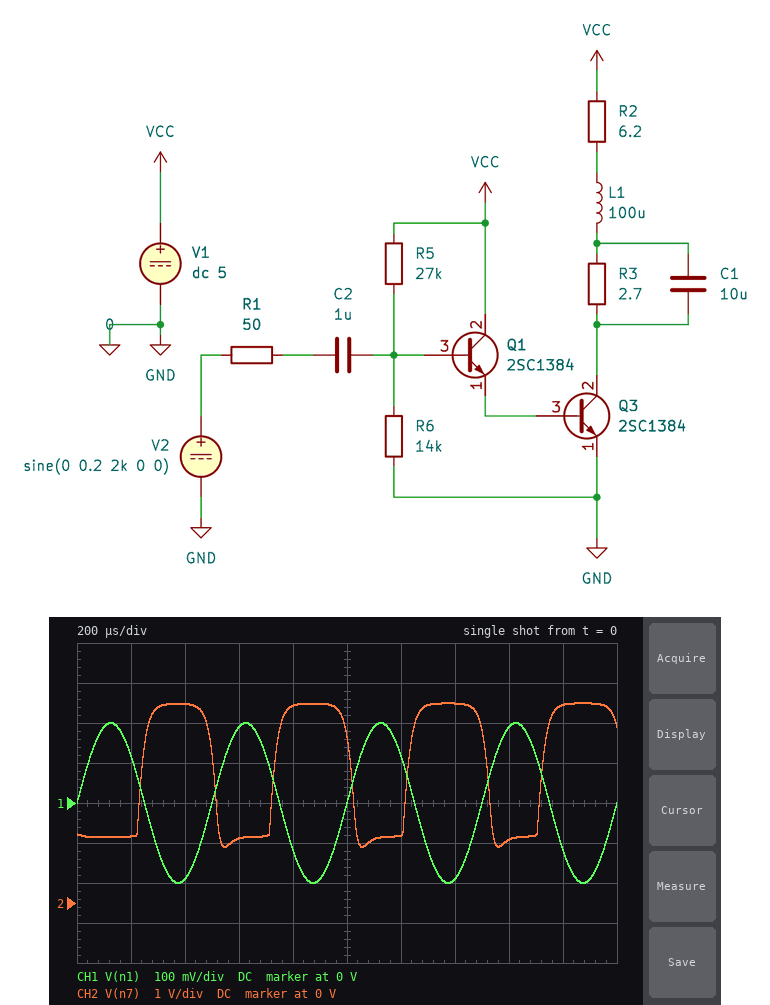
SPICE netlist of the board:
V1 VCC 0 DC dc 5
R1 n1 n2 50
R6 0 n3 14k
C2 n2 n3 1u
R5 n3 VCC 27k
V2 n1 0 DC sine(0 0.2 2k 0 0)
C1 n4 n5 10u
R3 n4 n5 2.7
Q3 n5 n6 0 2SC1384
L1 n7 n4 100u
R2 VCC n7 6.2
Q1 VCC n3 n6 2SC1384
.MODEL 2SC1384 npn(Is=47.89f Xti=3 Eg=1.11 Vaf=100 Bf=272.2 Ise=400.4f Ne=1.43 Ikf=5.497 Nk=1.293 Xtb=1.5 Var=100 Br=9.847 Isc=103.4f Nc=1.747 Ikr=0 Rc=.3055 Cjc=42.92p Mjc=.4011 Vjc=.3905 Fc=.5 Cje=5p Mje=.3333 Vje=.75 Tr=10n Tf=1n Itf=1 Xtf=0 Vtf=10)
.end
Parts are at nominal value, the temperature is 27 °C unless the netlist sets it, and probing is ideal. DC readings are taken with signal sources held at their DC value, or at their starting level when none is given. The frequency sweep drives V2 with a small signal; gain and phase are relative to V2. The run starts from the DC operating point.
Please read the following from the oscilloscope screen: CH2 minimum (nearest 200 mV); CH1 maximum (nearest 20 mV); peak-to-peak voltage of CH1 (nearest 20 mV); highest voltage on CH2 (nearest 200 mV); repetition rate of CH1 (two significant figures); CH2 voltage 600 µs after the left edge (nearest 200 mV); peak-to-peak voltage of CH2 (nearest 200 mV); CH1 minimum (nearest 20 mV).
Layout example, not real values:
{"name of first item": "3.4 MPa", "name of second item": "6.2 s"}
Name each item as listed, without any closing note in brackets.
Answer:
{"CH2 minimum": "1.4 V", "CH1 maximum": "200 mV", "peak-to-peak voltage of CH1": "400 mV", "highest voltage on CH2": "5.0 V", "repetition rate of CH1": "2.0 kHz", "CH2 voltage 600 µs after the left edge": "1.6 V", "peak-to-peak voltage of CH2": "3.6 V", "CH1 minimum": "-200 mV"}
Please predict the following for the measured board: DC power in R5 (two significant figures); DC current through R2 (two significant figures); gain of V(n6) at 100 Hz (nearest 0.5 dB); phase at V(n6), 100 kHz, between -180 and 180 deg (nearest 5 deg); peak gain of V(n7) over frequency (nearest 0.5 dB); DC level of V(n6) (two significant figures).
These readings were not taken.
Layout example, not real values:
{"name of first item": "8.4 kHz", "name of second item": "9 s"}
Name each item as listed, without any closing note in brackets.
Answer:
{"DC power in R5": "470 µW", "DC current through R2": "530 mA", "gain of V(n6) at 100 Hz": "-26.0 dB", "phase at V(n6), 100 kHz, between -180 and 180 deg": "-5 deg", "peak gain of V(n7) over frequency": "10.0 dB", "DC level of V(n6)": "780 mV"}
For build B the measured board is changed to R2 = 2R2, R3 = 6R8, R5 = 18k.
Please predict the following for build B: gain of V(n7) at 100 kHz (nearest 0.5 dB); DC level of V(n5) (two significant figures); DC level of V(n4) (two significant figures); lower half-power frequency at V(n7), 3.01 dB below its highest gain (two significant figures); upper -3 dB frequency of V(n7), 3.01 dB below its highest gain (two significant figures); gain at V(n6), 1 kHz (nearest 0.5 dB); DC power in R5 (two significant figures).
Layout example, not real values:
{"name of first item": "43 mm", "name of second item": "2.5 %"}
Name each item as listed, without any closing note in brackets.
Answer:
{"gain of V(n7) at 100 kHz": "-31.5 dB", "DC level of V(n5)": "220 mV", "DC level of V(n4)": "3.8 V", "lower half-power frequency at V(n7), 3.01 dB below its highest gain": "3.0 kHz", "upper -3 dB frequency of V(n7), 3.01 dB below its highest gain": "9.6 kHz", "gain at V(n6), 1 kHz": "-16.0 dB", "DC power in R5": "690 µW"}
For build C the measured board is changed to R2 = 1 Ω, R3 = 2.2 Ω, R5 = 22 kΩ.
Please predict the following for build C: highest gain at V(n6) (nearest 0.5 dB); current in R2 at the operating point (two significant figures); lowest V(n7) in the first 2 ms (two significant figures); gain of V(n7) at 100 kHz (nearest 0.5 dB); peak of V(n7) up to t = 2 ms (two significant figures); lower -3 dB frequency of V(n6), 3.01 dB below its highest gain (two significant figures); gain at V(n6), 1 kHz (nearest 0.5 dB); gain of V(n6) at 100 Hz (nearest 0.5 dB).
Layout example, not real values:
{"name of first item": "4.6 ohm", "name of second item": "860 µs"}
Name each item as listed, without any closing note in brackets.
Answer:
{"highest gain at V(n6)": "-6.0 dB", "current in R2 at the operating point": "1.1 A", "lowest V(n7) in the first 2 ms": "3.5 V", "gain of V(n7) at 100 kHz": "20.5 dB", "peak of V(n7) up to t = 2 ms": "5.0 V", "lower -3 dB frequency of V(n6), 3.01 dB below its highest gain": "170 Hz", "gain at V(n6), 1 kHz": "-6.5 dB", "gain of V(n6) at 100 Hz": "-11.5 dB"}
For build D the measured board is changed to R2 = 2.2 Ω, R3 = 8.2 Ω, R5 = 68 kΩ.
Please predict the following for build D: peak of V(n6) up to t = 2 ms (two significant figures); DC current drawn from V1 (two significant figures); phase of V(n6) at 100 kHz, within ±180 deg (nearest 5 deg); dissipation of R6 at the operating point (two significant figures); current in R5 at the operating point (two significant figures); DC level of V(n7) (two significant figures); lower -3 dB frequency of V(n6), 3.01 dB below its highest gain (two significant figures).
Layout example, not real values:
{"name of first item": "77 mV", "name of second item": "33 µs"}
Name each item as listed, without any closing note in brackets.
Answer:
{"peak of V(n6) up to t = 2 ms": "580 mV", "DC current drawn from V1": "65 µA", "phase of V(n6) at 100 kHz, within ±180 deg": "-25 deg", "dissipation of R6 at the operating point": "52 µW", "current in R5 at the operating point": "61 µA", "DC level of V(n7)": "5.0 V", "lower -3 dB frequency of V(n6), 3.01 dB below its highest gain": "5.6 MHz"}
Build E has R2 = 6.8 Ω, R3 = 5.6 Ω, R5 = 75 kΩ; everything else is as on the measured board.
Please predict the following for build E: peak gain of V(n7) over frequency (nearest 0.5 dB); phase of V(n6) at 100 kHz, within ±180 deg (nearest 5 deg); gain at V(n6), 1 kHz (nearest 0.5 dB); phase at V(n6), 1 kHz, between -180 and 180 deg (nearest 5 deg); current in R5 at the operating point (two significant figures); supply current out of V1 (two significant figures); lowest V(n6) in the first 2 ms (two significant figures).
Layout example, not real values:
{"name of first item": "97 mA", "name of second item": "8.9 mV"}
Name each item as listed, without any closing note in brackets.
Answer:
{"peak gain of V(n7) over frequency": "-39.5 dB", "phase of V(n6) at 100 kHz, within ±180 deg": "-15 deg", "gain at V(n6), 1 kHz": "-5.0 dB", "phase at V(n6), 1 kHz, between -180 and 180 deg": "0 deg", "current in R5 at the operating point": "56 µA", "supply current out of V1": "57 µA", "lowest V(n6) in the first 2 ms": "350 mV"}
